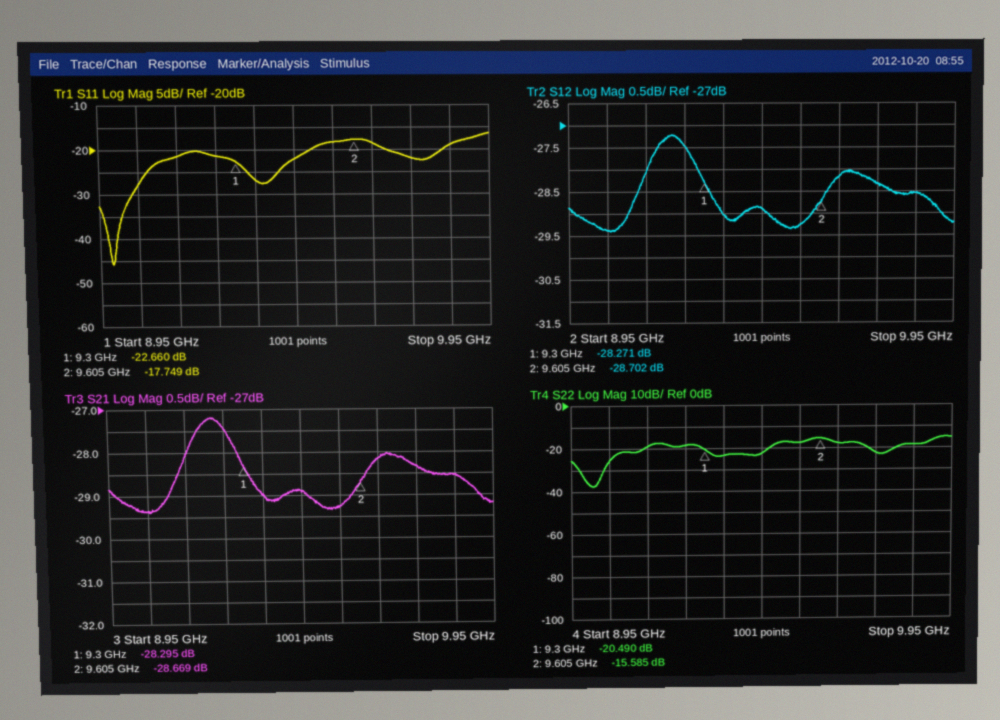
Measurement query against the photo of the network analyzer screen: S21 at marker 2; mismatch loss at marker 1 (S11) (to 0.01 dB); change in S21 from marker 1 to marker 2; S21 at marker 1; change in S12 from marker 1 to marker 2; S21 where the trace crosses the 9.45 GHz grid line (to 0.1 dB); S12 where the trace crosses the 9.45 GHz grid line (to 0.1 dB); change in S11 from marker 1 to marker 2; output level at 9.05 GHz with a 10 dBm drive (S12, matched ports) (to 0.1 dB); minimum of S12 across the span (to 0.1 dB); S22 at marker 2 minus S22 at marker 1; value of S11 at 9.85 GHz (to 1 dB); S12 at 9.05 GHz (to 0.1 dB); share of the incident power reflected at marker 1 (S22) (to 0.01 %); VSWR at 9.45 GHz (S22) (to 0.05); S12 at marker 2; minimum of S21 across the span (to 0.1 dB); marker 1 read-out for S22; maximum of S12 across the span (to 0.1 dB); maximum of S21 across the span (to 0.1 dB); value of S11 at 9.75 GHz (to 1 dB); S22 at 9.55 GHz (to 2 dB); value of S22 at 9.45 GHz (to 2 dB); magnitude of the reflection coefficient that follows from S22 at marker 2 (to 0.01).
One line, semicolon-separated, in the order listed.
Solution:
-28.669 dB; 0.02 dB; -0.374 dB; -28.295 dB; -0.431 dB; -28.9 dB; -28.9 dB; 4.911 dB; -19.4 dBm; -29.4 dB; 4.905 dB; -19 dB; -29.4 dB; 0.89 %; 1.15; -28.702 dB; -29.4 dB; -20.490 dB; -27.2 dB; -27.2 dB; -22 dB; -18 dB; -22 dB; 0.17
